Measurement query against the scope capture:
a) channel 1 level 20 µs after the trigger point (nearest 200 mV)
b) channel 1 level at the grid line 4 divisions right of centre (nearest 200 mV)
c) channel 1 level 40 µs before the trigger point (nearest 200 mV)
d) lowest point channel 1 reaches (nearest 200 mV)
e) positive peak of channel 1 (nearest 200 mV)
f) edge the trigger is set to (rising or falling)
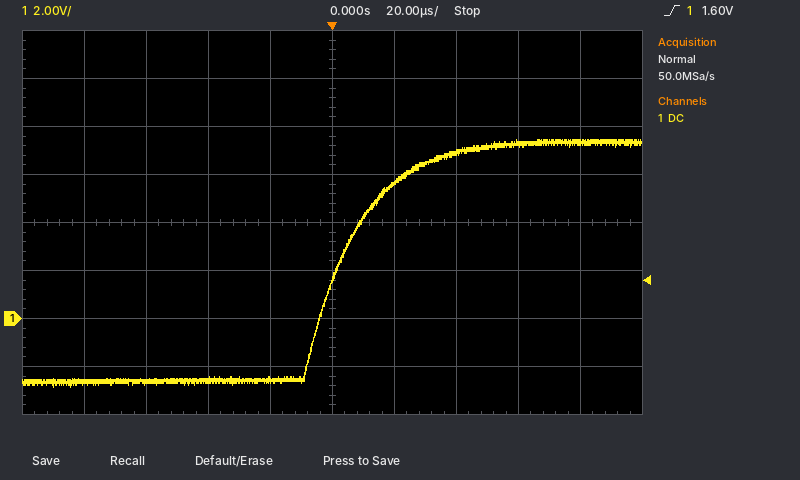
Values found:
5.6 V
7.4 V
-2.6 V
-2.8 V
7.4 V
rising
